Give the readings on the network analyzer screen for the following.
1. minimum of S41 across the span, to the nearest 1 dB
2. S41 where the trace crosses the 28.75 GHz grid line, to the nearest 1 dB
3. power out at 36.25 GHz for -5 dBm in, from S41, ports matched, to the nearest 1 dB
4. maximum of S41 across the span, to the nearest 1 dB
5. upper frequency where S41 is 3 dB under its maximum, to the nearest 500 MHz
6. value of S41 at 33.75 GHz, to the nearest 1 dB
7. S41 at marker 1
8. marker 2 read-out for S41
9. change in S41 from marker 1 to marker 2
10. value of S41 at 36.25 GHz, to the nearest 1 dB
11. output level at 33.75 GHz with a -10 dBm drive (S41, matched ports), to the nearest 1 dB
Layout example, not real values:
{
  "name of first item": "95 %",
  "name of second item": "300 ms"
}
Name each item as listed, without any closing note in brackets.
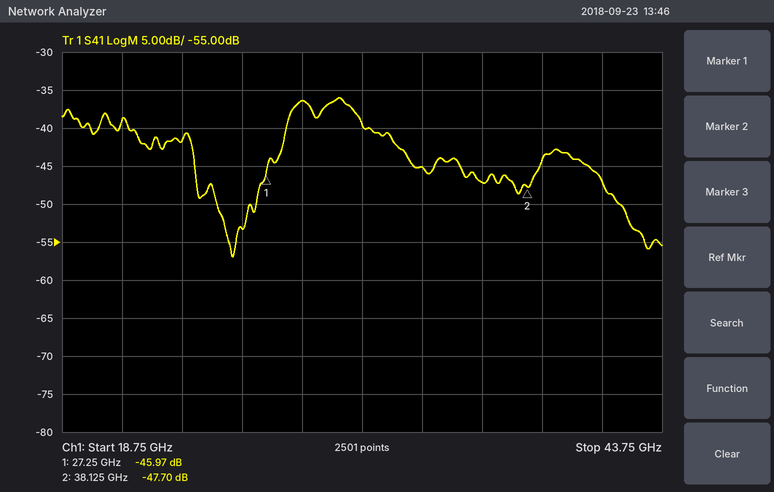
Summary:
{
  "minimum of S41 across the span, to the nearest 1 dB": "-57 dB",
  "S41 where the trace crosses the 28.75 GHz grid line, to the nearest 1 dB": "-36 dB",
  "power out at 36.25 GHz for -5 dBm in, from S41, ports matched, to the nearest 1 dB": "-52 dBm",
  "maximum of S41 across the span, to the nearest 1 dB": "-36 dB",
  "upper frequency where S41 is 3 dB under its maximum, to the nearest 500 MHz": "31.0 GHz",
  "value of S41 at 33.75 GHz, to the nearest 1 dB": "-45 dB",
  "S41 at marker 1": "-45.97 dB",
  "marker 2 read-out for S41": "-47.70 dB",
  "change in S41 from marker 1 to marker 2": "-1.73 dB",
  "value of S41 at 36.25 GHz, to the nearest 1 dB": "-47 dB",
  "output level at 33.75 GHz with a -10 dBm drive (S41, matched ports), to the nearest 1 dB": "-55 dBm"
}
